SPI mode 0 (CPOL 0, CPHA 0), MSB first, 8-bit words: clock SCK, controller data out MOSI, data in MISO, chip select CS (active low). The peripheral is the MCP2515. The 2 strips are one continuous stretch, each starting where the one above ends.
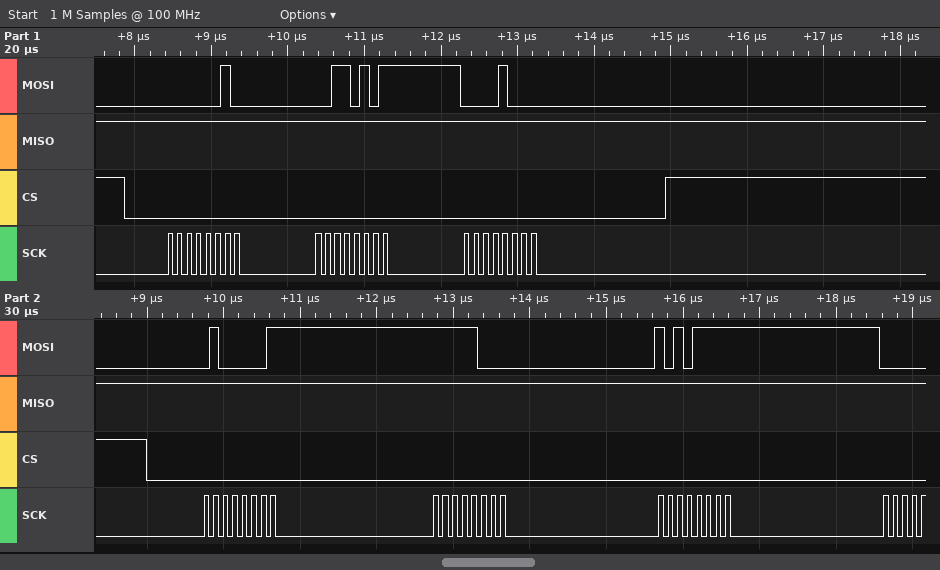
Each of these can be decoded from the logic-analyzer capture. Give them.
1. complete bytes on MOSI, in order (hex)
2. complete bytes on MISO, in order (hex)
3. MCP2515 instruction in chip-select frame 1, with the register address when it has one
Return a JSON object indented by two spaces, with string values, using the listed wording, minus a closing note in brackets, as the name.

{
  "complete bytes on MOSI, in order": "0x02 0x35 0x08 0x41 0xF8 0xAF",
  "complete bytes on MISO, in order": "0xFF 0xFF 0xFF 0xFF 0xFF 0xFF",
  "MCP2515 instruction in chip-select frame 1, with the register address when it has one": "WRITE 0x35"
}
